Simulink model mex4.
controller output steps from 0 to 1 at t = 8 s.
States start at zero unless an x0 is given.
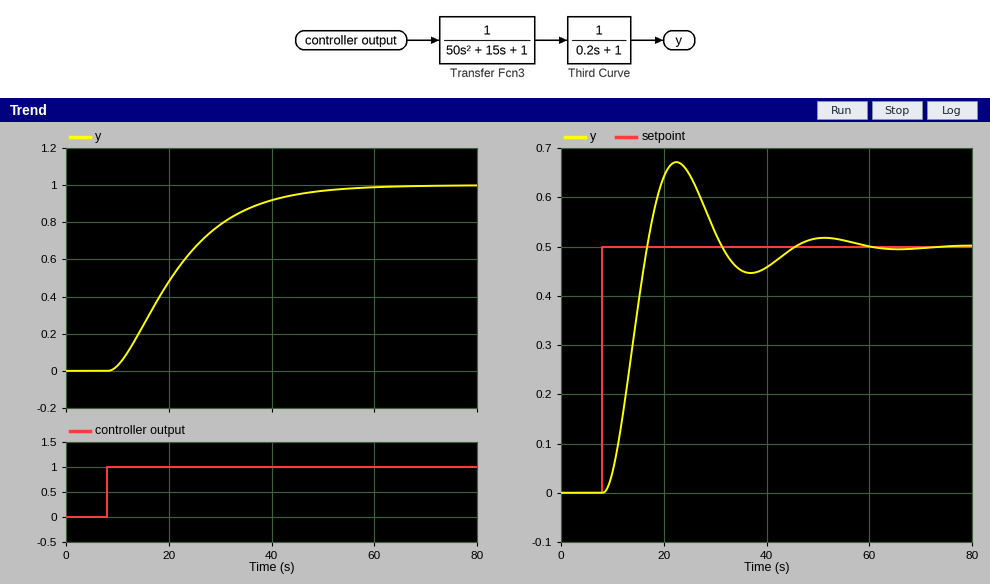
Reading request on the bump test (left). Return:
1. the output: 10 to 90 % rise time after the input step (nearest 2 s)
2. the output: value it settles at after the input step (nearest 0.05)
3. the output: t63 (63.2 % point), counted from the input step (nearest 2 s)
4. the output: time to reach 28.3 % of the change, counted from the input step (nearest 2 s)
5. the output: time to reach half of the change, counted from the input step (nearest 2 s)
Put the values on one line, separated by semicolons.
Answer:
26 s; 1.00; 16 s; 8 s; 12 s
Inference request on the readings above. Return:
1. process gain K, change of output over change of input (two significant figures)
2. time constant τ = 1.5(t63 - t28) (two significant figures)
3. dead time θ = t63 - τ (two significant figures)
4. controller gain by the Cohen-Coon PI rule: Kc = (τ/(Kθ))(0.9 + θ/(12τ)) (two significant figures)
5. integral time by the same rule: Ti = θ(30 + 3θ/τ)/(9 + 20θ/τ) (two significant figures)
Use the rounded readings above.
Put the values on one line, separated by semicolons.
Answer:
1.0; 12 s; 4.0 s; 2.8; 7.9 s
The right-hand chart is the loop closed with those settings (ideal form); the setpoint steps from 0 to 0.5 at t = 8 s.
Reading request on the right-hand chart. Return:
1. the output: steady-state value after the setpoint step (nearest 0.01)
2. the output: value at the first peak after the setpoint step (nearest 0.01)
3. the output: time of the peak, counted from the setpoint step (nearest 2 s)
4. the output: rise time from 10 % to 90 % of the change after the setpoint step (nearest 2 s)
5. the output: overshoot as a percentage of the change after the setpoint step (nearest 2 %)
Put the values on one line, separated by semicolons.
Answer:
0.50; 0.67; 14 s; 6 s; 34 %
